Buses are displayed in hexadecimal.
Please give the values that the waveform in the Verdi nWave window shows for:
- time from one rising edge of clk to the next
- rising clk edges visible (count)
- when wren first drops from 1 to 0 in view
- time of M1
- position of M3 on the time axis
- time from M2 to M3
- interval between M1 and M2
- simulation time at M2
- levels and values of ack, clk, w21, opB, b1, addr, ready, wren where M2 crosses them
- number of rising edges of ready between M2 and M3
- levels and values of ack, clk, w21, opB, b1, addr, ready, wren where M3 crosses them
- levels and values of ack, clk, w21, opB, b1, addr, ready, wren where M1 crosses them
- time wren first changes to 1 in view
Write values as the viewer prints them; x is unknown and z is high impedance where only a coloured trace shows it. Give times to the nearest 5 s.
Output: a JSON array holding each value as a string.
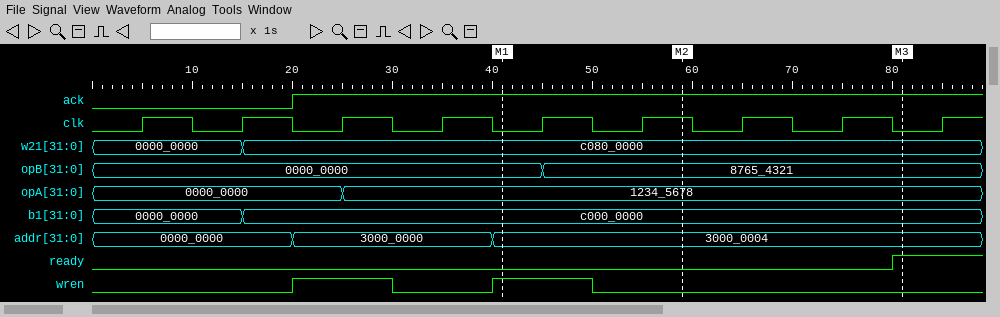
["10 s", "9", "30 s", "40 s", "80 s", "20 s", "20 s", "60 s", "ack=1, clk=1, w21=c080_0000, opB=8765_4321, b1=c000_0000, addr=3000_0004, ready=0, wren=0", "1", "ack=1, clk=0, w21=c080_0000, opB=8765_4321, b1=c000_0000, addr=3000_0004, ready=1, wren=0", "ack=1, clk=0, w21=c080_0000, opB=0000_0000, b1=c000_0000, addr=3000_0004, ready=0, wren=1", "20 s"]
